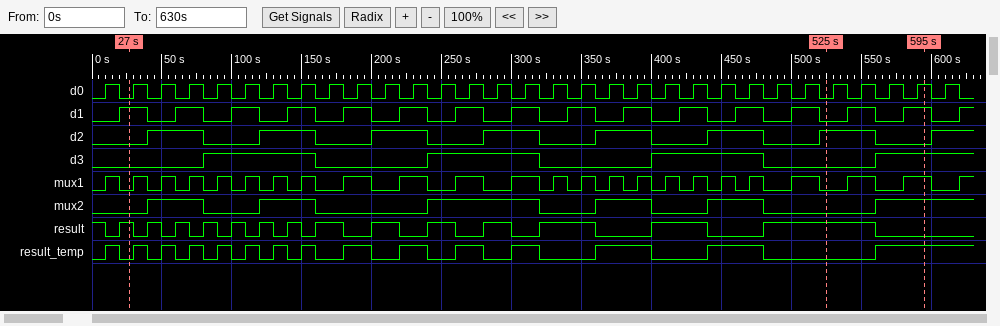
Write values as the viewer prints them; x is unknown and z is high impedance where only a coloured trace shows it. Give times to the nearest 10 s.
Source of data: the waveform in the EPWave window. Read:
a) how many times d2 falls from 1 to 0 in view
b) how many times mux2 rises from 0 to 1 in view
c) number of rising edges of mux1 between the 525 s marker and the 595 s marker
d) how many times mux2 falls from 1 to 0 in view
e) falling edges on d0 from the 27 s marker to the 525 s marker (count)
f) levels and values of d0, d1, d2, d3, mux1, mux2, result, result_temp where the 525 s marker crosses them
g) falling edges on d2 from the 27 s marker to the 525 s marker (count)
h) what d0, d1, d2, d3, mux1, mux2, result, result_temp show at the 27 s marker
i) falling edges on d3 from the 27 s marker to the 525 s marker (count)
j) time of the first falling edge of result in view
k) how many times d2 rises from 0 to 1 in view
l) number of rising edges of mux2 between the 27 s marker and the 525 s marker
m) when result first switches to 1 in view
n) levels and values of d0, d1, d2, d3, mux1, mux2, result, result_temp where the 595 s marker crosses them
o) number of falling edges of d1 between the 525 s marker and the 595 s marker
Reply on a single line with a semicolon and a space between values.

7; 6; 2; 5; 25; d0=0, d1=0, d2=1, d3=0, mux1=0, mux2=0, result=1, result_temp=0; 6; d0=0, d1=1, d2=0, d3=0, mux1=0, mux2=0, result=1, result_temp=0; 3; 10 s; 8; 5; 20 s; d0=1, d1=1, d2=0, d3=1, mux1=1, mux2=1, result=0, result_temp=1; 1
